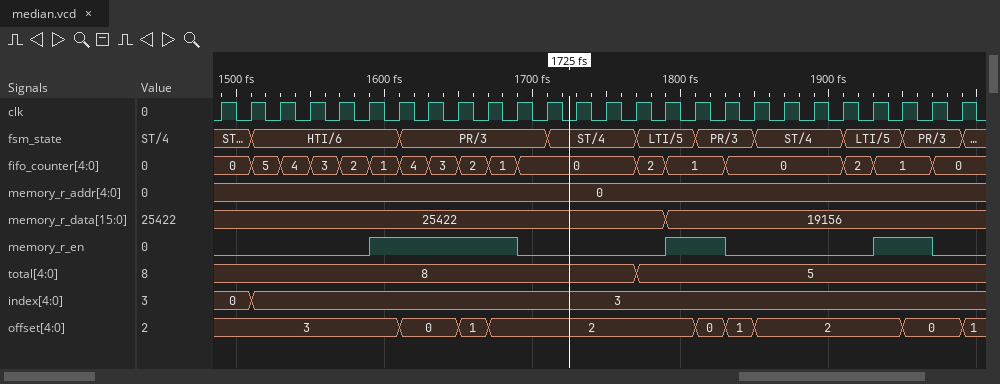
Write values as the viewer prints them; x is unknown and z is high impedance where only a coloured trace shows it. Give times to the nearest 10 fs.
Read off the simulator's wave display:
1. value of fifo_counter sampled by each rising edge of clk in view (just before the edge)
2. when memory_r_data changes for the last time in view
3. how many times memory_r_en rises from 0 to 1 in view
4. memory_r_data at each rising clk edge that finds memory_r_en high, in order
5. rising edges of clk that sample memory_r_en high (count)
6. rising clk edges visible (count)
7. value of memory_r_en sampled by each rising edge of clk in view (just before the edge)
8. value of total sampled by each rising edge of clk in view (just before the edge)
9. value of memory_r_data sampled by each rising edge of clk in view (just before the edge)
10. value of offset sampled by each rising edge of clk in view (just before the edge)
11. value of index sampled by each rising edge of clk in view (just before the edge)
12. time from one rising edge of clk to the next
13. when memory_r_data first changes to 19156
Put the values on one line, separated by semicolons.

0, 0, 5, 4, 3, 2, 1, 4, 3, 2, 1, 0, 0, 0, 0, 2, 1, 1, 0, 0, 0, 0, 2, 1, 1, 0; 1790 fs; 3; 25422, 25422, 25422, 25422, 25422, 19156, 19156, 19156, 19156; 9; 26; 0 0 0 0 0 0 1 1 1 1 1 0 0 0 0 0 1 1 0 0 0 0 0 1 1 0; 8, 8, 8, 8, 8, 8, 8, 8, 8, 8, 8, 8, 8, 8, 8, 5, 5, 5, 5, 5, 5, 5, 5, 5, 5, 5; 25422, 25422, 25422, 25422, 25422, 25422, 25422, 25422, 25422, 25422, 25422, 25422, 25422, 25422, 25422, 25422, 19156, 19156, 19156, 19156, 19156, 19156, 19156, 19156, 19156, 19156; 3, 3, 3, 3, 3, 3, 3, 0, 0, 1, 2, 2, 2, 2, 2, 2, 2, 0, 1, 2, 2, 2, 2, 2, 0, 0; 0, 0, 3, 3, 3, 3, 3, 3, 3, 3, 3, 3, 3, 3, 3, 3, 3, 3, 3, 3, 3, 3, 3, 3, 3, 3; 20 fs; 1790 fs
